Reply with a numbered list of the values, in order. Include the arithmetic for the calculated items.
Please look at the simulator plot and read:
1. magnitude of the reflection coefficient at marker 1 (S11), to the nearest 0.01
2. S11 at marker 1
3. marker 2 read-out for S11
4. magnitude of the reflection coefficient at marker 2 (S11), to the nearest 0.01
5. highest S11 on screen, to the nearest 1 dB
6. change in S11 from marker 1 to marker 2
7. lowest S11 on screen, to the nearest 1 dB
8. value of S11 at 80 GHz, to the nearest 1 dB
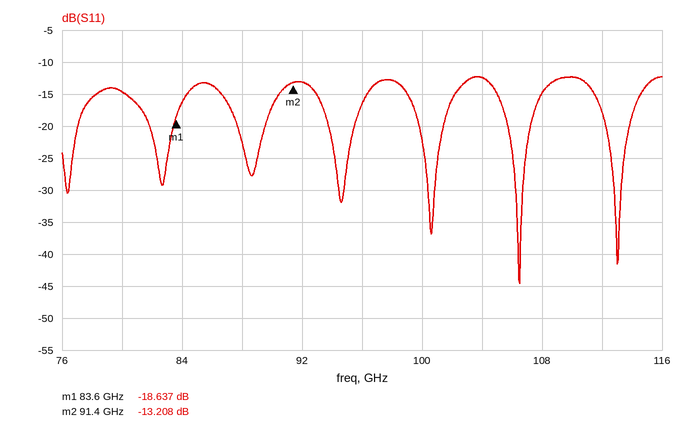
1. 10^(-18.637/20) ≈ 0.12
2. -18.637 dB
3. -13.208 dB
4. 10^(-13.208/20) ≈ 0.22
5. -12 dB
6. -13.208 − (-18.637) = 5.429 dB
7. -45 dB
8. -15 dB
